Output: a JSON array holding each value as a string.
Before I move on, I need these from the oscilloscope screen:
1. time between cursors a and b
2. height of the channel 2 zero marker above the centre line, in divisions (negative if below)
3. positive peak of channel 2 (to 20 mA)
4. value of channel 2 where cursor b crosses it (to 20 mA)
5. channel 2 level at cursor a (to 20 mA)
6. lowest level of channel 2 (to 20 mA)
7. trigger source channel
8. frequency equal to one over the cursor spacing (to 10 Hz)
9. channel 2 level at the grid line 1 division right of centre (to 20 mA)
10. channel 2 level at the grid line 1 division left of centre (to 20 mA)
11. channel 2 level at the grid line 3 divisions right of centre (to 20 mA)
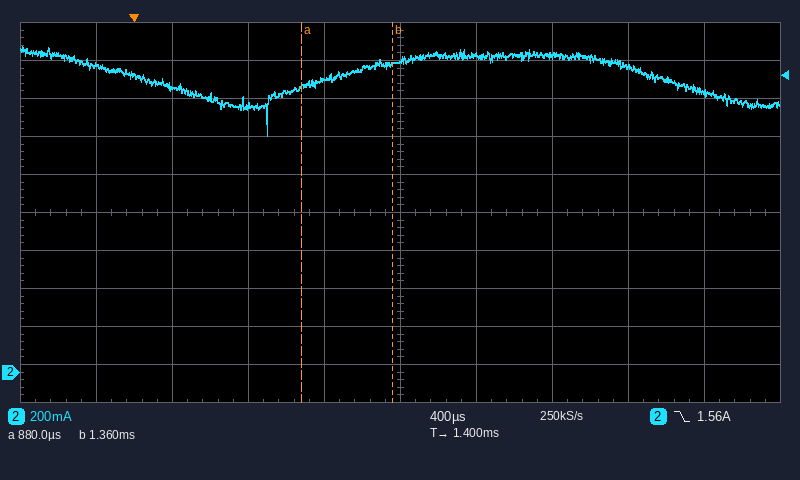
["480 µs", "-4.2 div", "1.72 A", "1.62 A", "1.50 A", "1.24 A", "channel 2", "2.08 kHz", "1.66 A", "1.54 A", "1.60 A"]
